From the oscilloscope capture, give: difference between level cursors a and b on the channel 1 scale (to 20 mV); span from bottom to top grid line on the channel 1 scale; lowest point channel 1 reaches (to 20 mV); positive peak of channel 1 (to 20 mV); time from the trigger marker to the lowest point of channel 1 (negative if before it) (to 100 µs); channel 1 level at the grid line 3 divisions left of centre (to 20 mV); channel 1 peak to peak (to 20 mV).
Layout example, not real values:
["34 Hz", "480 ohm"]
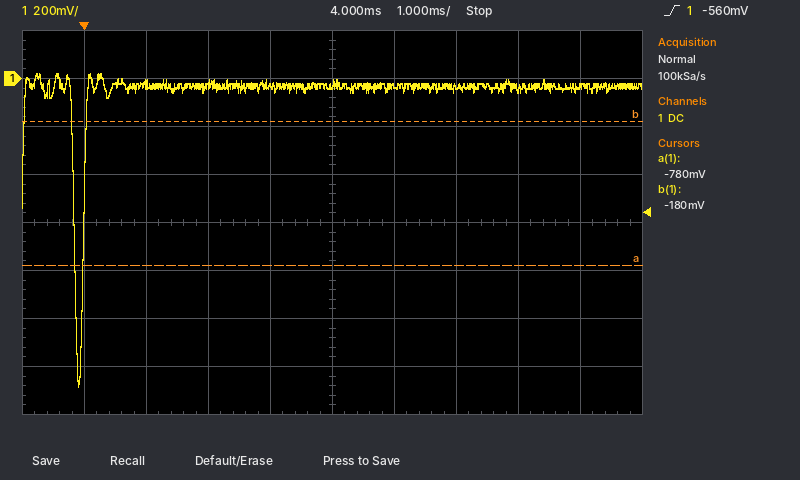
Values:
["600 mV", "1.6 V", "-1.28 V", "20 mV", "-100 µs", "-20 mV", "1.30 V"]
